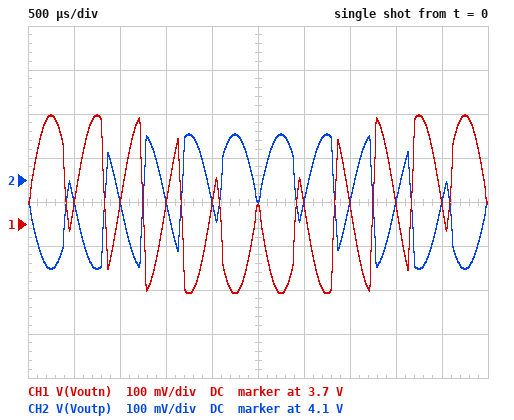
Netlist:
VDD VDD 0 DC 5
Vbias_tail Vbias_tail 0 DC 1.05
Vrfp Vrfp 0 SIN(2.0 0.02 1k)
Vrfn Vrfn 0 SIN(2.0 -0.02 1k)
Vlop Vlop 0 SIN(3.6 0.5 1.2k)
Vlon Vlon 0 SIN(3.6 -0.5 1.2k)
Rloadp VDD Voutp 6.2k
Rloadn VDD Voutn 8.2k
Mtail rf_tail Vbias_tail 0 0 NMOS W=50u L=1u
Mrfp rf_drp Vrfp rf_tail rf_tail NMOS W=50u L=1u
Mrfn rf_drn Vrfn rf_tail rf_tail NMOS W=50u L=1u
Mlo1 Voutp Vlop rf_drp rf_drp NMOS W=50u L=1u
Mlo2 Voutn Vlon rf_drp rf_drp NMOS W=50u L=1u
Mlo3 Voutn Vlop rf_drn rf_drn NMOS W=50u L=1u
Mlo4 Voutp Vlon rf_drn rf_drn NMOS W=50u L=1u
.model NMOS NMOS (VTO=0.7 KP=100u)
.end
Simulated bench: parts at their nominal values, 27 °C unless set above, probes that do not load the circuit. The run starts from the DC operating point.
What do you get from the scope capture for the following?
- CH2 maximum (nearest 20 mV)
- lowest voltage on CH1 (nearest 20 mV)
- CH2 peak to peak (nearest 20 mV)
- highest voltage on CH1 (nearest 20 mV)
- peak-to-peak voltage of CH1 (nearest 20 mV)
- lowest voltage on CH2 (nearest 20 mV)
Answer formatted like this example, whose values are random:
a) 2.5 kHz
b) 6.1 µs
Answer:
a) 4.20 V
b) 3.54 V
c) 300 mV
d) 3.94 V
e) 400 mV
f) 3.90 V
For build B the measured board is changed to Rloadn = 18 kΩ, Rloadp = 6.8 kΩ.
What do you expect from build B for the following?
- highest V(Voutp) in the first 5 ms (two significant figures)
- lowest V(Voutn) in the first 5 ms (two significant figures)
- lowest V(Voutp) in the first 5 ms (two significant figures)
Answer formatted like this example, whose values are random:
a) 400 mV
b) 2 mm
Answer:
a) 3.9 V
b) 2.5 V
c) 3.7 V
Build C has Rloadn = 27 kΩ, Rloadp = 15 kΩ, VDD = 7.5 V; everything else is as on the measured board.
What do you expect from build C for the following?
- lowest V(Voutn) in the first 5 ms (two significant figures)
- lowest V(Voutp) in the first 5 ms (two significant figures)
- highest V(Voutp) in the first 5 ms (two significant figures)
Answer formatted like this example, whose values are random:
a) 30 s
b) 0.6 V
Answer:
a) 2.7 V
b) 4.8 V
c) 5.6 V
